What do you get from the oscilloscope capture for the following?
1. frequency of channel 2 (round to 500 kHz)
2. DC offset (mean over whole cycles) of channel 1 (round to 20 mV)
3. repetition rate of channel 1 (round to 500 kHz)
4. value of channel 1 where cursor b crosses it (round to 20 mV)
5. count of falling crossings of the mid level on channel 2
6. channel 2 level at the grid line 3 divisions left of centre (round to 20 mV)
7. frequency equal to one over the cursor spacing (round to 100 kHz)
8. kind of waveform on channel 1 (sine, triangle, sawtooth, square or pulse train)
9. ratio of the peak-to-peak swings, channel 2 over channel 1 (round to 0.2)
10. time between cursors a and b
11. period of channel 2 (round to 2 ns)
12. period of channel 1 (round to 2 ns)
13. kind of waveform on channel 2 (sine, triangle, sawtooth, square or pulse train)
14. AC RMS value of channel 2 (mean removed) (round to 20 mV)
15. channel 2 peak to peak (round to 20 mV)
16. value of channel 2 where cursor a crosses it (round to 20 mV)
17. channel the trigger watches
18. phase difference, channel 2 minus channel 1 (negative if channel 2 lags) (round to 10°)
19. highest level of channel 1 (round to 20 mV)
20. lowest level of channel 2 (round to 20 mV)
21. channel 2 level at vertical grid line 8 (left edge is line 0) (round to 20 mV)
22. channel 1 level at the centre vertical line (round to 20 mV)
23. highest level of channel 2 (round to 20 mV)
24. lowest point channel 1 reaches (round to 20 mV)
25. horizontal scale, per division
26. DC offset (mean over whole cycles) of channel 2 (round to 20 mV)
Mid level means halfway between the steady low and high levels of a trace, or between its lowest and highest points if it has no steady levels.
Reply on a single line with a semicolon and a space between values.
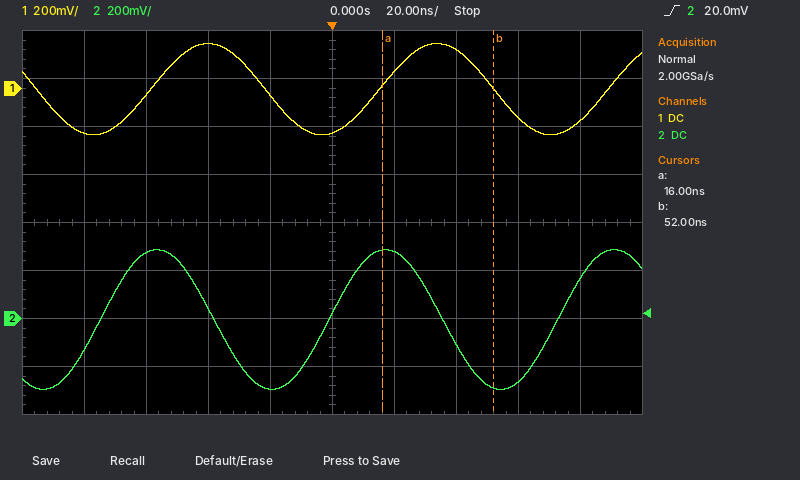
13.5 MHz; 0 mV; 13.5 MHz; 0 mV; 2; 280 mV; 27.8 MHz; sine; 1.6; 36 ns; 74 ns; 74 ns; sine; 200 mV; 580 mV; 280 mV; channel 2; +80°; 180 mV; -300 mV; -260 mV; -180 mV; 280 mV; -200 mV; 20 ns; 0 mV
